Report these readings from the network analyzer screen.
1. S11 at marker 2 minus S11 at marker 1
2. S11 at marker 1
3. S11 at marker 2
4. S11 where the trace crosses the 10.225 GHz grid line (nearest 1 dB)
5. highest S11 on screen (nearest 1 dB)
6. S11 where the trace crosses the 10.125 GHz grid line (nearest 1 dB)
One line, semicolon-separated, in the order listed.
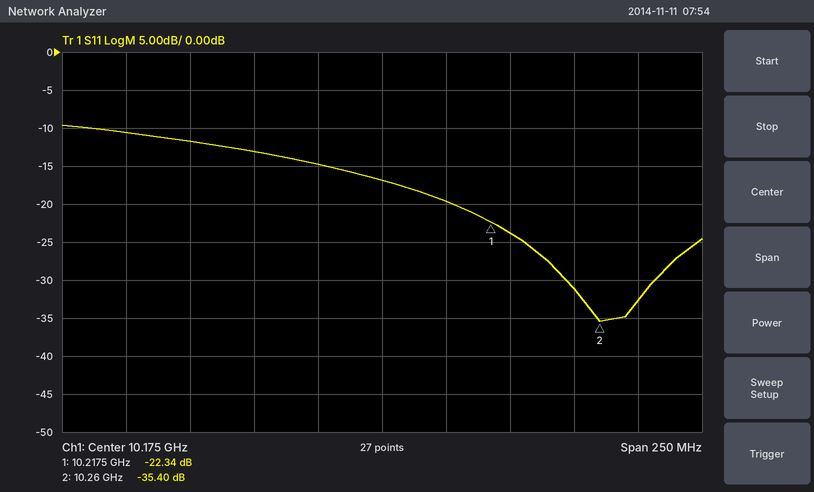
-13.06 dB; -22.34 dB; -35.40 dB; -24 dB; -10 dB; -13 dB
